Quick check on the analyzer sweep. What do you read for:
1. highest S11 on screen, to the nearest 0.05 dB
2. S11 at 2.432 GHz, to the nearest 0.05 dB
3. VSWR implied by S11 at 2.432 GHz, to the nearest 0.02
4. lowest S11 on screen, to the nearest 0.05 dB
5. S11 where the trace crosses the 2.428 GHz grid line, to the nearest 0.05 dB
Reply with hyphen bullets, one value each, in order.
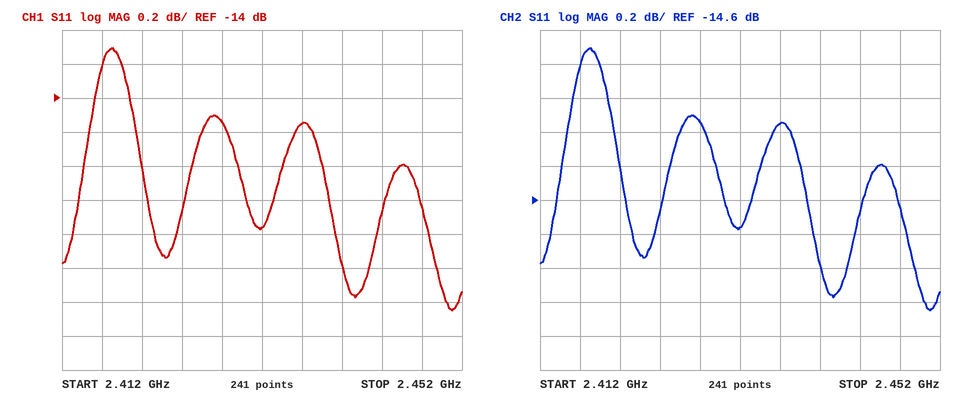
- -13.70 dB
- -14.75 dB
- 1.44
- -15.25 dB
- -14.15 dB
